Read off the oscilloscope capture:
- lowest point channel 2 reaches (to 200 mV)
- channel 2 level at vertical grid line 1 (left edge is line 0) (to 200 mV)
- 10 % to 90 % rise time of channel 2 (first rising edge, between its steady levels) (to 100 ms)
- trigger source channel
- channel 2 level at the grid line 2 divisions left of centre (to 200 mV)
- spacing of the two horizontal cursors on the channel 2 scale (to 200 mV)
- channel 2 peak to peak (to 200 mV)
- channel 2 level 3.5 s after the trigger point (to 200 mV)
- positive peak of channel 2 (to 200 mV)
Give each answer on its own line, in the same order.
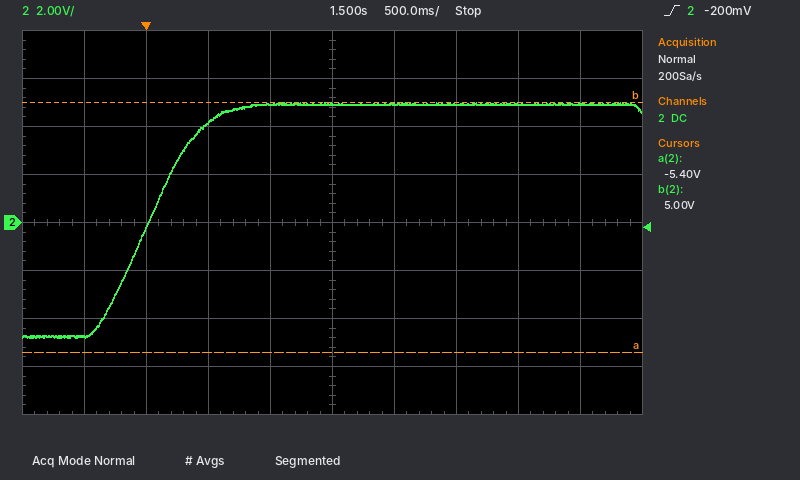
-4.8 V
-4.8 V
800 ms
channel 2
4.2 V
10.4 V
9.8 V
5.0 V
5.0 V
